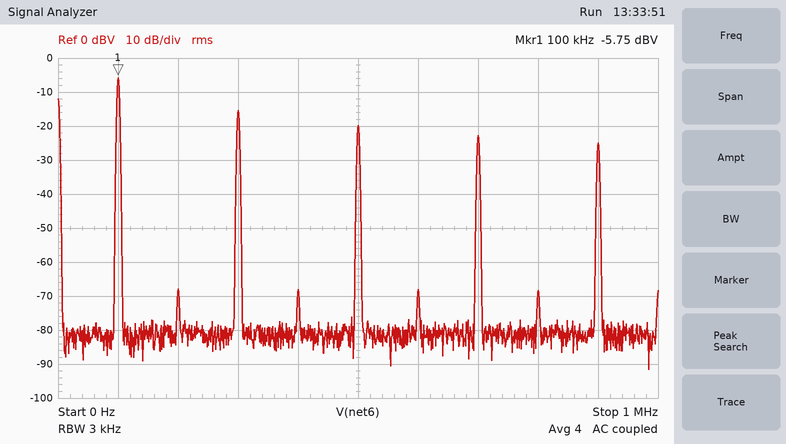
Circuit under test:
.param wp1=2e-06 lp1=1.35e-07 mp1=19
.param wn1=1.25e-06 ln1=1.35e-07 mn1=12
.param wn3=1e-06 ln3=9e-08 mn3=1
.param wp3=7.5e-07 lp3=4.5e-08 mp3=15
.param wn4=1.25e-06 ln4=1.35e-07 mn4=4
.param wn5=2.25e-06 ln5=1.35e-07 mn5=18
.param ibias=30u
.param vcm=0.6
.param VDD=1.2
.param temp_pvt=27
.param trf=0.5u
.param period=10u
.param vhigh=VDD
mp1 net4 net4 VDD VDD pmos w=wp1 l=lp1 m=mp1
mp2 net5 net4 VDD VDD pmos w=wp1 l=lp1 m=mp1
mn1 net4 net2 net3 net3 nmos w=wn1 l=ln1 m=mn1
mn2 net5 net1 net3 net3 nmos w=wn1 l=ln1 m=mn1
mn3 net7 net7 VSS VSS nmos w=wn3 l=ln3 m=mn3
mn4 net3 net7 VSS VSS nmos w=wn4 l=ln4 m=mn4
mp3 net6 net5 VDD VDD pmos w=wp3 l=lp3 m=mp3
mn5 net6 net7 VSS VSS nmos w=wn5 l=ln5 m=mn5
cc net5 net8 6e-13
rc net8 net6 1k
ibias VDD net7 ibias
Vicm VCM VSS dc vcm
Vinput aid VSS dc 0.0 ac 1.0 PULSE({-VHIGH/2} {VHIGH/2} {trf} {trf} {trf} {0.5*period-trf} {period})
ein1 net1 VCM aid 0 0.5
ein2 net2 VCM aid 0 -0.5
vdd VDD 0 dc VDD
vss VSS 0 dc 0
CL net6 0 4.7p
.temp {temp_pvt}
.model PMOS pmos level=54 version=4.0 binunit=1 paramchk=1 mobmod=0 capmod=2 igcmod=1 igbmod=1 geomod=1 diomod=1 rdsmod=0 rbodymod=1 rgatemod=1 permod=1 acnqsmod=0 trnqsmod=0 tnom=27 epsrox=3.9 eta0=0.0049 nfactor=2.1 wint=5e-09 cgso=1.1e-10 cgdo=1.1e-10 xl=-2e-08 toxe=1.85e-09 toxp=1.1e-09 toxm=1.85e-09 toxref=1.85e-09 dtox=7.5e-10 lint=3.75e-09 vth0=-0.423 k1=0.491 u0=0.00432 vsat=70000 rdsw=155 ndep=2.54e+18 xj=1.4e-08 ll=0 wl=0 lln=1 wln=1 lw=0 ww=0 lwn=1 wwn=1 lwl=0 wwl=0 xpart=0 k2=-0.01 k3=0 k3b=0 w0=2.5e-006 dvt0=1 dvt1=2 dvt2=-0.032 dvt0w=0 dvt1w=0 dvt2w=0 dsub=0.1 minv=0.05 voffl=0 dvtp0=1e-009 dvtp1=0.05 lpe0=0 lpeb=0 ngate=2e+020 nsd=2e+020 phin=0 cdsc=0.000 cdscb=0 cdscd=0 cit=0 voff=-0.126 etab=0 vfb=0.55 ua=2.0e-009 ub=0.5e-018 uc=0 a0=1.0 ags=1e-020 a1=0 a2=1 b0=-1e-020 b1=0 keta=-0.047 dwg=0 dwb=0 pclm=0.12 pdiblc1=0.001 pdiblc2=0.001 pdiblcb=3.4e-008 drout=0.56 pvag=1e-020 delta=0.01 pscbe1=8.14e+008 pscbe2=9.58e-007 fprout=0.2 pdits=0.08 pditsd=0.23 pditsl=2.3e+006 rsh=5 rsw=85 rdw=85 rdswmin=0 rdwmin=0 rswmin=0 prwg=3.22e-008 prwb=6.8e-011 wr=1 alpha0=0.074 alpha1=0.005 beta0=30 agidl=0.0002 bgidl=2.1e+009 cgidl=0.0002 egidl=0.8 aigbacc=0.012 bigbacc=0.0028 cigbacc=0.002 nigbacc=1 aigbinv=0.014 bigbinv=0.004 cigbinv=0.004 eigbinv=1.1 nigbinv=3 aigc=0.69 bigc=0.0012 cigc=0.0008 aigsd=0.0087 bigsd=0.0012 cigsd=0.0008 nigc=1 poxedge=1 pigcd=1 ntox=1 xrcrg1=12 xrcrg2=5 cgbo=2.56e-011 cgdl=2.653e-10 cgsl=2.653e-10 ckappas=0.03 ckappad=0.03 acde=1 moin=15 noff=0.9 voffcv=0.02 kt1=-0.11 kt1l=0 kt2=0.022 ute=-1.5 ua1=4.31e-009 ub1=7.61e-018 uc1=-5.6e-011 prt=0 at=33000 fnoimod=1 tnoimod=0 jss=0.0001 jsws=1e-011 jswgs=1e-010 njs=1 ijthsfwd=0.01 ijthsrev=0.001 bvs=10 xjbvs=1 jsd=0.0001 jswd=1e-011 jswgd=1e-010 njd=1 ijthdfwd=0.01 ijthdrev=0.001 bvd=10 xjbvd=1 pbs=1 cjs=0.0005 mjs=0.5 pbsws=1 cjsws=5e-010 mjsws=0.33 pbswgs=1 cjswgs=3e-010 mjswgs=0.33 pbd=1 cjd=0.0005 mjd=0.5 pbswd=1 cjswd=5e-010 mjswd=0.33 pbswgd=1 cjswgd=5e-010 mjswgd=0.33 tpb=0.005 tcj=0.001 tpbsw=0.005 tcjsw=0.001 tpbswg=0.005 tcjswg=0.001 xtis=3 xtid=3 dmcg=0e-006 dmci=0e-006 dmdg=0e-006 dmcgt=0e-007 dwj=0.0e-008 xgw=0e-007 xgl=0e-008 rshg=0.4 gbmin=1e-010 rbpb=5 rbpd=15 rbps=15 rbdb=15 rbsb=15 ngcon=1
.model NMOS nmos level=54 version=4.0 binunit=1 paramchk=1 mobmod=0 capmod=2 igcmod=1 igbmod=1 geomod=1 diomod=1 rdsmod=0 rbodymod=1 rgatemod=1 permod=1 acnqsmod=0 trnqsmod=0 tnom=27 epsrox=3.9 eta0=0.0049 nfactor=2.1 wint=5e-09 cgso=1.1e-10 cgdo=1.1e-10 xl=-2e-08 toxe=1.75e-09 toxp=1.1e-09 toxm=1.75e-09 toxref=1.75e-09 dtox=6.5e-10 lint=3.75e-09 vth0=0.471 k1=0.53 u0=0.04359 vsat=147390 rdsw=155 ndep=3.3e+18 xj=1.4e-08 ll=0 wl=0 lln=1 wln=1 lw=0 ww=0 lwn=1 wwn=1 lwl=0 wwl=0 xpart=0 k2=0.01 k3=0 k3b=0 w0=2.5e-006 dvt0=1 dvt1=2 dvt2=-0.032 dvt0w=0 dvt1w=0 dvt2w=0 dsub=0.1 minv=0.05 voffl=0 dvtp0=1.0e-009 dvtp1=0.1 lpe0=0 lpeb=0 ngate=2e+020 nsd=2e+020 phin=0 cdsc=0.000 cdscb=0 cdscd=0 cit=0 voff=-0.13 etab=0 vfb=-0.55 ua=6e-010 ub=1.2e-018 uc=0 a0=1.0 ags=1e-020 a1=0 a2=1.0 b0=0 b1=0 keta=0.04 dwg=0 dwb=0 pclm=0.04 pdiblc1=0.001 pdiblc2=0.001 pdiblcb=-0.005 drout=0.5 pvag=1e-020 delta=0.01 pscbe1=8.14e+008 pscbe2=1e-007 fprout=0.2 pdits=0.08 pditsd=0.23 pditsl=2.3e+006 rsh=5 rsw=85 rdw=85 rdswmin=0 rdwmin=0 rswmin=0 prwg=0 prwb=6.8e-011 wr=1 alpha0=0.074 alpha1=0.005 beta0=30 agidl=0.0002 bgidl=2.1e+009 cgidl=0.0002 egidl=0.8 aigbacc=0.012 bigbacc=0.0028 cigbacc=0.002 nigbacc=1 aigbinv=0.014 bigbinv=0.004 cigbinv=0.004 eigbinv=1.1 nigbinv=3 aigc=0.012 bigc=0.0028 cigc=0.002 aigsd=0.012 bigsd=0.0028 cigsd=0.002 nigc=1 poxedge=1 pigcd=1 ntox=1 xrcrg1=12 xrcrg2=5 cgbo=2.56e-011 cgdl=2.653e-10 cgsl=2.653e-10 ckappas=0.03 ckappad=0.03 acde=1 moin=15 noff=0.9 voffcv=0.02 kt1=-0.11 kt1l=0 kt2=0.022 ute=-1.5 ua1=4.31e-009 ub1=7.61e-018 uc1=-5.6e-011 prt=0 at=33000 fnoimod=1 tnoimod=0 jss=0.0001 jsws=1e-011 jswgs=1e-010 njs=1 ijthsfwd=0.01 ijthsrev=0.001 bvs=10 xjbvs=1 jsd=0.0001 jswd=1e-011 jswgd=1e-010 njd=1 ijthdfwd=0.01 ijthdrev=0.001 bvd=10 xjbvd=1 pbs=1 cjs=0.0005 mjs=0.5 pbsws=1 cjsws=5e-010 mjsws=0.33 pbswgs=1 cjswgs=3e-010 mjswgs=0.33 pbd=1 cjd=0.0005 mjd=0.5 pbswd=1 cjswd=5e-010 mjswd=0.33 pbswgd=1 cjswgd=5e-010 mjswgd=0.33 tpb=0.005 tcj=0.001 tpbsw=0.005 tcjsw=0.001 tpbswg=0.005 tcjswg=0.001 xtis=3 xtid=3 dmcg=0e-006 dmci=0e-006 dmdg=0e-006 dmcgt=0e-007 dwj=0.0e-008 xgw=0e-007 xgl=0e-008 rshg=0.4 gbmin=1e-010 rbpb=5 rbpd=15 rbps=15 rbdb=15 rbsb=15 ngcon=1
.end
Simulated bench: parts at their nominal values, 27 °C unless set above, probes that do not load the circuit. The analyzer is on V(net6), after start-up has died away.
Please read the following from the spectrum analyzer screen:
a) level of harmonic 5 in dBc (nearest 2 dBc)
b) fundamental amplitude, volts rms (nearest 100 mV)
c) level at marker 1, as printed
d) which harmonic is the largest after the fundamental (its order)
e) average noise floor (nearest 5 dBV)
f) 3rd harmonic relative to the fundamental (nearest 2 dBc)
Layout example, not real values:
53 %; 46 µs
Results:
-14 dBc; 500 mV; -5.75 dBV; 3; -80 dBV; -10 dBc
